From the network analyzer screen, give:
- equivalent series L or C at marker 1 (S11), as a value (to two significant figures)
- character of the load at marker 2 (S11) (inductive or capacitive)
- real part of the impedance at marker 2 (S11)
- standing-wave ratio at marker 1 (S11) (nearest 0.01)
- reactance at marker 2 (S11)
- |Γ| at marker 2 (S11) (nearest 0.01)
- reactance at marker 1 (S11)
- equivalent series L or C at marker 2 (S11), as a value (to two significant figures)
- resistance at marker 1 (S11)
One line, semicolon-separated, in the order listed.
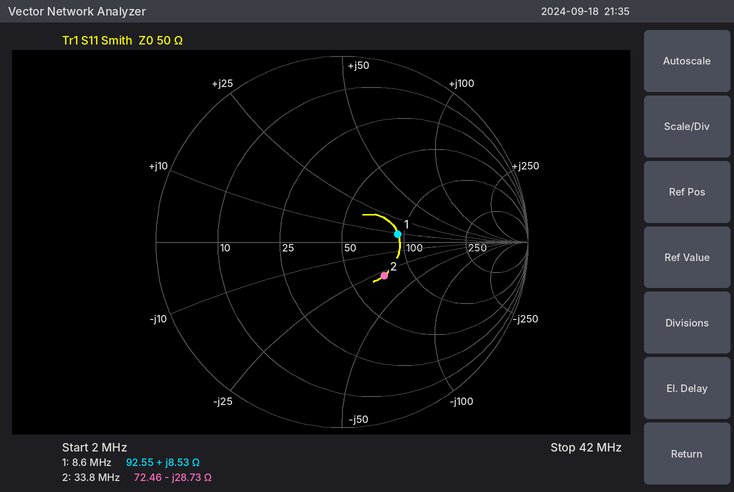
160 nH; capacitive; 72.46 Ω; 1.87; -28.73 Ω; 0.29; +8.53 Ω; 160 pF; 92.55 Ω
